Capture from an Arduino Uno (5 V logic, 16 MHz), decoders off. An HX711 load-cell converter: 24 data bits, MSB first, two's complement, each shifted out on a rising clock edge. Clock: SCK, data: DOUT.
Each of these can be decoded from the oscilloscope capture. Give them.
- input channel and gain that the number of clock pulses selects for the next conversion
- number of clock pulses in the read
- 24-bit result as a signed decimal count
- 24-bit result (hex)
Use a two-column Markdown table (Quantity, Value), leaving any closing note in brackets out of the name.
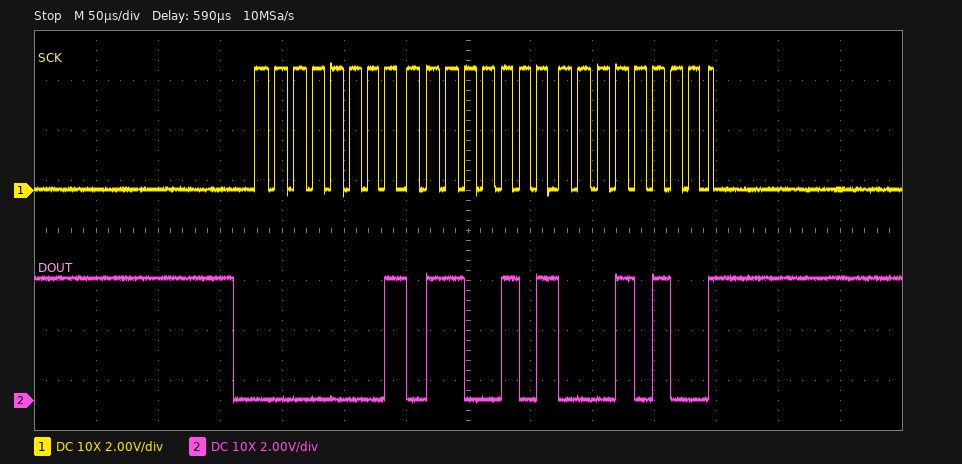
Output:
| Quantity | Value |
|---|---|
| input channel and gain that the number of clock pulses selects for the next conversion | channel A, gain 128 |
| number of clock pulses in the read | 25 |
| 24-bit result as a signed decimal count | 91412 |
| 24-bit result | 0x016514 |
